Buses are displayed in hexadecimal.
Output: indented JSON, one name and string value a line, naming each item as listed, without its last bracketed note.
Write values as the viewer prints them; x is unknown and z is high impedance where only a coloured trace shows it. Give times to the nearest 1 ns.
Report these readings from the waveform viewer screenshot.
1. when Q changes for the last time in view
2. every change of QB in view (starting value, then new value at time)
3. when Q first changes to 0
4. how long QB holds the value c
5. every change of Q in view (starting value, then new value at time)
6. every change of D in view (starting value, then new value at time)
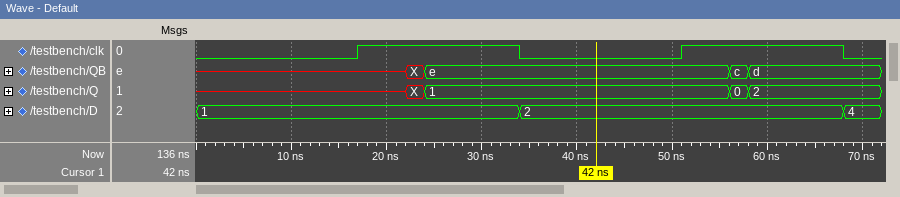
{
  "when Q changes for the last time in view": "58 ns",
  "every change of QB in view": "x, X at 22 ns, e at 24 ns, c at 56 ns, d at 58 ns",
  "when Q first changes to 0": "56 ns",
  "how long QB holds the value c": "2 ns",
  "every change of Q in view": "x, X at 22 ns, 1 at 24 ns, 0 at 56 ns, 2 at 58 ns",
  "every change of D in view": "1, 2 at 34 ns, 4 at 68 ns"
}
